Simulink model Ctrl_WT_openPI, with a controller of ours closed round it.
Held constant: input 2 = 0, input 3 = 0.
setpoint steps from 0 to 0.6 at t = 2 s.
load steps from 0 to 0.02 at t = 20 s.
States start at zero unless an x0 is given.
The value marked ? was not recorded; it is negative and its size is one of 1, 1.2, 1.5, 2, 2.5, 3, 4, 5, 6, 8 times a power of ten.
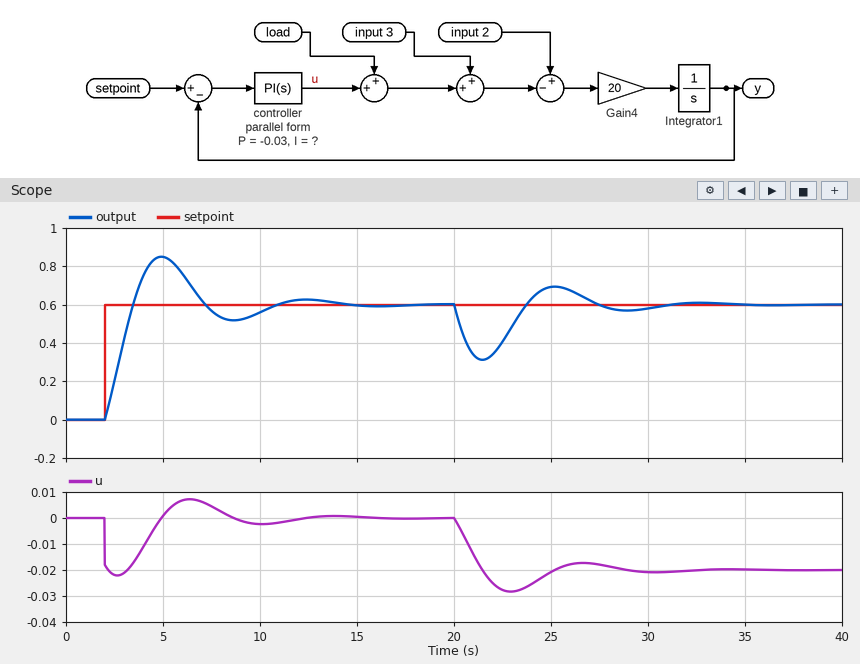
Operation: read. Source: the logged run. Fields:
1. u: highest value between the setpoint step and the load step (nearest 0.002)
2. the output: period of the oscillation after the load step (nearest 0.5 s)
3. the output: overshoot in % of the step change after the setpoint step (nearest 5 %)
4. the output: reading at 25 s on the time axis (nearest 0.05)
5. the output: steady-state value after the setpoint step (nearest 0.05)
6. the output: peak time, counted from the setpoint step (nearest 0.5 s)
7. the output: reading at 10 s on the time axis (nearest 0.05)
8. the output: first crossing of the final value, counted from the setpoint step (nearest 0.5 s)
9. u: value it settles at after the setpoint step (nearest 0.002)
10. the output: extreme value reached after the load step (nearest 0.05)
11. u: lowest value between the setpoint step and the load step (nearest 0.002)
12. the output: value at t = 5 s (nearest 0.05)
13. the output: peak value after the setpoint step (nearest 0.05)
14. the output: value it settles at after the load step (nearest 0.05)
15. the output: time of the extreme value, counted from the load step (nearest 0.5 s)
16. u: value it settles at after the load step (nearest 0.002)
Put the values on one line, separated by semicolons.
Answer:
0.008; 7.5 s; 40 %; 0.70; 0.60; 3.0 s; 0.55; 1.5 s; 0.000; 0.30; -0.022; 0.85; 0.85; 0.60; 1.5 s; -0.020
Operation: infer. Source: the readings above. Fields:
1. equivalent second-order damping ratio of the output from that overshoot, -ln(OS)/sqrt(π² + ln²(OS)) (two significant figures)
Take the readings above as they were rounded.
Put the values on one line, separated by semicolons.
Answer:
0.28
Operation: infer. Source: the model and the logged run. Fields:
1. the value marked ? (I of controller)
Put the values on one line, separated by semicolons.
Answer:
-0.04
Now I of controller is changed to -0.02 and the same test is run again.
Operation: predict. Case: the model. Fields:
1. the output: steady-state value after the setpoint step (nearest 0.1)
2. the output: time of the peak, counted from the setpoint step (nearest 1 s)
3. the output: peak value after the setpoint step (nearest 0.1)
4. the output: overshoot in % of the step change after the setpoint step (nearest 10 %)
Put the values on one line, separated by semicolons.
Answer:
0.6; 4 s; 0.8; 30 %
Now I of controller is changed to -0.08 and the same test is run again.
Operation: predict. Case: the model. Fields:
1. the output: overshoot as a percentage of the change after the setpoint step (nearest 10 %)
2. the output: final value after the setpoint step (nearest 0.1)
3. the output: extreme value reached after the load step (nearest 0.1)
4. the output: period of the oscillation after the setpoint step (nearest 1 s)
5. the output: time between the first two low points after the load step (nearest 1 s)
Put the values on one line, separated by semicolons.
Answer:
50 %; 0.6; 0.4; 5 s; 5 s
